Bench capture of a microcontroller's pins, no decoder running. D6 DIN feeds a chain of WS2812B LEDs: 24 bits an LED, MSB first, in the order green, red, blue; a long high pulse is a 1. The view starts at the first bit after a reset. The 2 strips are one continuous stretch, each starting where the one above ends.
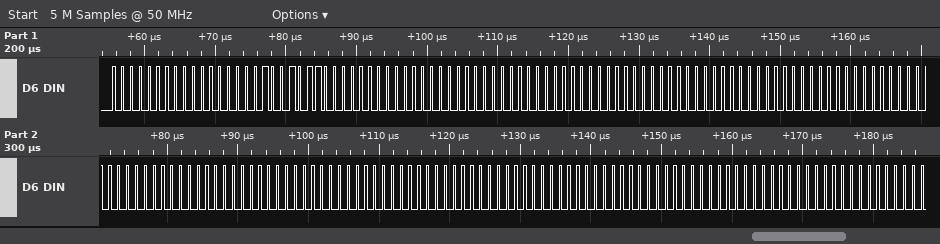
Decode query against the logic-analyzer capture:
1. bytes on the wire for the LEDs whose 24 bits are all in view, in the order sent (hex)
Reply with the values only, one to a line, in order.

00 00 4B 00 00 00 00 00 00 00 00 00 00 00 00 00 00 00 00 00 00
